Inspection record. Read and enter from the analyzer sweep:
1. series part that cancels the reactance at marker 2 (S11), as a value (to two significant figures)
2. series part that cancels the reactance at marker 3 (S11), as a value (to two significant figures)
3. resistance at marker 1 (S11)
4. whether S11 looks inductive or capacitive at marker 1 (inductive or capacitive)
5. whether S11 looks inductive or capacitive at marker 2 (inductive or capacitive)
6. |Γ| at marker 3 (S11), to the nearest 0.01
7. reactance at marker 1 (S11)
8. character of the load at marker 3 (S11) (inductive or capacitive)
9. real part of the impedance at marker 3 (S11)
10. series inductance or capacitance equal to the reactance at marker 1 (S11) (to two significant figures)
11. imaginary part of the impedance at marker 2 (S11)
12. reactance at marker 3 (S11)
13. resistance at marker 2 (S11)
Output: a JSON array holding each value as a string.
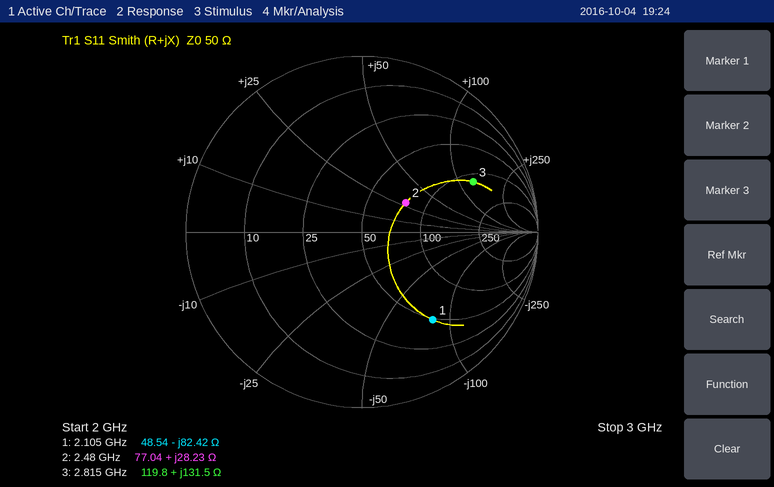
["2.3 pF", "430 fF", "48.54 Ω", "capacitive", "inductive", "0.69", "-82.42 Ω", "inductive", "119.8 Ω", "920 fF", "+28.23 Ω", "+131.5 Ω", "77.04 Ω"]
